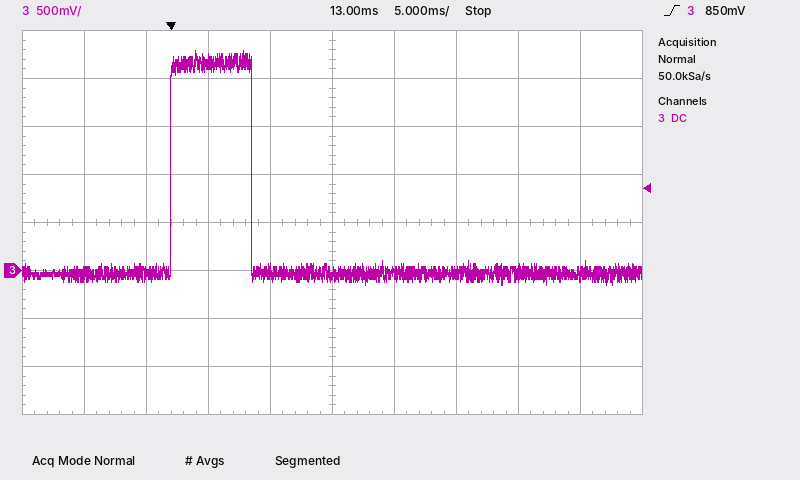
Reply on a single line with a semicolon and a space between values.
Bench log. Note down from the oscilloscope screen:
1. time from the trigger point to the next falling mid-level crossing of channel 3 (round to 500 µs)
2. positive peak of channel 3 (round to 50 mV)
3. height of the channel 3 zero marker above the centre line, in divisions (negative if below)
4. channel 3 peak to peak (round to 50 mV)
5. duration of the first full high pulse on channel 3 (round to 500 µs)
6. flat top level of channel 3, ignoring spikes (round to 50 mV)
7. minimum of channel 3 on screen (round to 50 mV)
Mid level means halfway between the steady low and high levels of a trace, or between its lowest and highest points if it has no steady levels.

6.5 ms; 2.30 V; -1.0 div; 2.45 V; 6.5 ms; 2.15 V; -150 mV
